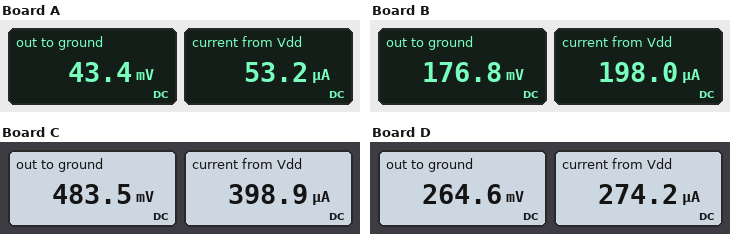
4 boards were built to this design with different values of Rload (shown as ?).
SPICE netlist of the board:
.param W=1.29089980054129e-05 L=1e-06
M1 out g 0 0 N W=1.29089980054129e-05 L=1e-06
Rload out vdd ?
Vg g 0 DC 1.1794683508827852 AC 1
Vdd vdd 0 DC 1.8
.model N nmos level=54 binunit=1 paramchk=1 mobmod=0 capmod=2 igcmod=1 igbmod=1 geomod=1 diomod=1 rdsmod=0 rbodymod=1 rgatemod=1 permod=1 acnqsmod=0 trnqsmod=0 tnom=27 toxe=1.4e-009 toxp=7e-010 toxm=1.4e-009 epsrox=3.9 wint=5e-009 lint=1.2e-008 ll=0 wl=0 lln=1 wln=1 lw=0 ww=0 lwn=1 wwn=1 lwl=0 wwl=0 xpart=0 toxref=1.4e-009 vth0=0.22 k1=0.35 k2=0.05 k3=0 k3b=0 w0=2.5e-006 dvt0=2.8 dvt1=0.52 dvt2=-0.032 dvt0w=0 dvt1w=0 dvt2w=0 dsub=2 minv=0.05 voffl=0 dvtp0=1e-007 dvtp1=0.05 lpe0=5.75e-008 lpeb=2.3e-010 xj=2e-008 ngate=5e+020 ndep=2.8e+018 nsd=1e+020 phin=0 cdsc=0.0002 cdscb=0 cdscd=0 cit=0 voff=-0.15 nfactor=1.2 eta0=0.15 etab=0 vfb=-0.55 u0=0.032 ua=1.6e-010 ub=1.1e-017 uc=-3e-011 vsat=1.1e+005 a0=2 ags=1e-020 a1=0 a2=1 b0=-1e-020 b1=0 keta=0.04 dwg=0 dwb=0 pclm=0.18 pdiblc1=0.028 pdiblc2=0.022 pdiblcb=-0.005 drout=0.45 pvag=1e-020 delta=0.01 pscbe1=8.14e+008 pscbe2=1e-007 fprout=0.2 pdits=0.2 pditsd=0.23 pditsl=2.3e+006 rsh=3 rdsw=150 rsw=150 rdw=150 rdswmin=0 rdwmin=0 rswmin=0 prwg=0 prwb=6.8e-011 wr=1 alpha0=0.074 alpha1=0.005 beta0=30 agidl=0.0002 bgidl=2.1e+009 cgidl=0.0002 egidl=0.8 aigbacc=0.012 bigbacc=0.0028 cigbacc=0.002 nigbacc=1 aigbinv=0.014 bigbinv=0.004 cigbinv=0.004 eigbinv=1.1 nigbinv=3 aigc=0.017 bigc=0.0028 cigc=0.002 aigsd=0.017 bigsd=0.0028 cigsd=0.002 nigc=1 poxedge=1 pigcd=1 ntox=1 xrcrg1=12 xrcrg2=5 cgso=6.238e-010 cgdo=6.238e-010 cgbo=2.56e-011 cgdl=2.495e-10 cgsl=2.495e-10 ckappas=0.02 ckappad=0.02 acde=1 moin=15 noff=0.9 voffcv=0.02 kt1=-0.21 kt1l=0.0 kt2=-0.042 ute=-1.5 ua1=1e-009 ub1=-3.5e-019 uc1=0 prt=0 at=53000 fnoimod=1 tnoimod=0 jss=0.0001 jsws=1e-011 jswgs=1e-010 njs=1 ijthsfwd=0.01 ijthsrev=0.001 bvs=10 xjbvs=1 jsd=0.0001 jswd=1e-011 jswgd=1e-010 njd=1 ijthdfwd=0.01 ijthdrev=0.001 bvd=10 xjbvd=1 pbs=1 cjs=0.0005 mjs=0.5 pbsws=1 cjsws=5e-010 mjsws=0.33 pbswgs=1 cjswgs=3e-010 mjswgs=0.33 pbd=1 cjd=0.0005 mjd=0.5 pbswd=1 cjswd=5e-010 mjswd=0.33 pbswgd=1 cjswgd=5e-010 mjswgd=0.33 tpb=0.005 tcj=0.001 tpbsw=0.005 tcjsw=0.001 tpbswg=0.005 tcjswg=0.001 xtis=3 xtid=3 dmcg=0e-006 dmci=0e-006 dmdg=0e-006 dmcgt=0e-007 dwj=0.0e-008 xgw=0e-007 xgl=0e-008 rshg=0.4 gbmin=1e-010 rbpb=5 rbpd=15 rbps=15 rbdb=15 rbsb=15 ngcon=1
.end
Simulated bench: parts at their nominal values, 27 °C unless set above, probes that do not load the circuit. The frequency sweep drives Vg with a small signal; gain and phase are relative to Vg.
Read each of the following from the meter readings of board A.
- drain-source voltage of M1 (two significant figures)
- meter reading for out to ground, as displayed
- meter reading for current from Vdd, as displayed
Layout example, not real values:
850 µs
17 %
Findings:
43 mV
43.4 mV
53.2 µA
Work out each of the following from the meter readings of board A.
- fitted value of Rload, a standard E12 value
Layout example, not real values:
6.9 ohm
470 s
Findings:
33 kΩ
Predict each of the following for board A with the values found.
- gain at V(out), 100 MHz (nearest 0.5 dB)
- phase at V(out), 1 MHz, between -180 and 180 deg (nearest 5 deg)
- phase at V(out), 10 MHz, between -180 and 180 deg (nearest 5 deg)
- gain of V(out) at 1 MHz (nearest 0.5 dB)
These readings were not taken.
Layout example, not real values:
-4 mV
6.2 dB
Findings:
-17.5 dB
10 deg
60 deg
-42.0 dB
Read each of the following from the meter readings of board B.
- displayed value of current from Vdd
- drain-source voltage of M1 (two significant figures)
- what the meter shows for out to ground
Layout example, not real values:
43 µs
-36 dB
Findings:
198.0 µA
180 mV
176.8 mV
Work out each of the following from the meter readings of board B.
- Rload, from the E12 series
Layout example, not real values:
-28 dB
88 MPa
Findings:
8.2 kΩ
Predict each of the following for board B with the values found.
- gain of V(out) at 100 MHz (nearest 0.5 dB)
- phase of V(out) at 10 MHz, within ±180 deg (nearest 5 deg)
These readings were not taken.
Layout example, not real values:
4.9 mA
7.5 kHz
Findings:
-16.5 dB
105 deg
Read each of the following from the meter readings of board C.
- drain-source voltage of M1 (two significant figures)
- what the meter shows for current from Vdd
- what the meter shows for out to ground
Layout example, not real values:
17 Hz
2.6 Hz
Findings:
480 mV
398.9 µA
483.5 mV
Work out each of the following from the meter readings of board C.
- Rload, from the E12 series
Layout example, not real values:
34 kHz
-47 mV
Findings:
3.3 kΩ
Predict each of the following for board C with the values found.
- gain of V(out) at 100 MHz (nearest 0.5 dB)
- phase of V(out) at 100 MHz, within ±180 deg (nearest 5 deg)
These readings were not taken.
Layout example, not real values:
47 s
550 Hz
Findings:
-10.0 dB
145 deg
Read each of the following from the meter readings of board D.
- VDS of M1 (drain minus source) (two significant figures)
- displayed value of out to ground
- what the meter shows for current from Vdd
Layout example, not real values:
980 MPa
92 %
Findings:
260 mV
264.6 mV
274.2 µA
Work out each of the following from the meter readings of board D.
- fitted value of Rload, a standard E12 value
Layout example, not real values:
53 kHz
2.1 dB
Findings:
5.6 kΩ
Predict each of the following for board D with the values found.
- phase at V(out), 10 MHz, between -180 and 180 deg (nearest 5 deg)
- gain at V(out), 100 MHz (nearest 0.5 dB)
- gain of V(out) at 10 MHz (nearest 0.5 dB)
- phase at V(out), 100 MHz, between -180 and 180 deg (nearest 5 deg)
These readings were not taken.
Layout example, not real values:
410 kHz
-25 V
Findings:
155 deg
-16.0 dB
-28.0 dB
95 deg
